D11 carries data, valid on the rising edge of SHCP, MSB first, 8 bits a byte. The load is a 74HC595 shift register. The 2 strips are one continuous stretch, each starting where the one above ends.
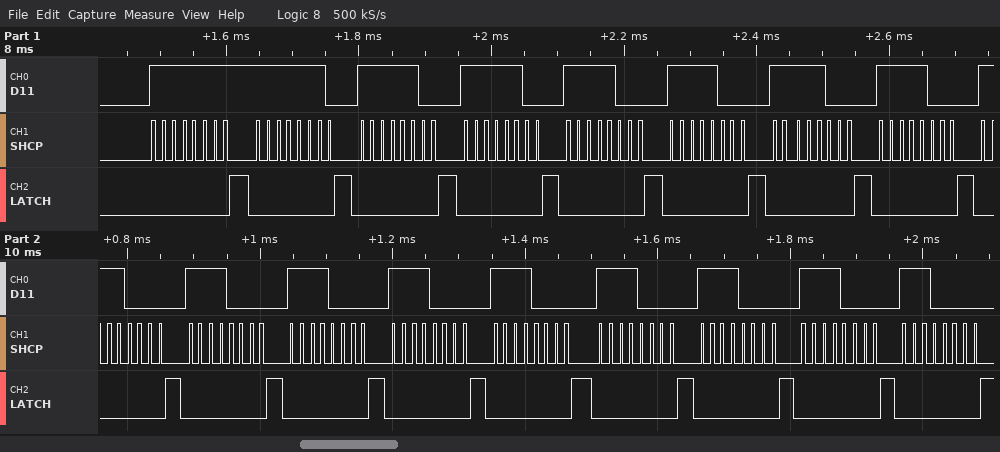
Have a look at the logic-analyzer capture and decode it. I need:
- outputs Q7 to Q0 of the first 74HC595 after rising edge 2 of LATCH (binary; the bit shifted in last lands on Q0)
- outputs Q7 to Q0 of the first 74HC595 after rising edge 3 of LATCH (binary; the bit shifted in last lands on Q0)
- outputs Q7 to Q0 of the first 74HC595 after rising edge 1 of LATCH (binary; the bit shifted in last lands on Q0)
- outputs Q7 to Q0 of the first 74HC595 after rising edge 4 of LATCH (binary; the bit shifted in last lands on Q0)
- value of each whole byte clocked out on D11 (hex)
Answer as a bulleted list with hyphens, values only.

- 11111110
- 11111100
- 11111111
- 11111100
- FF FE FC FC F8 F8 F8 F8 F0 F0 F0 F0 F0 F0 F0 F0 E0
